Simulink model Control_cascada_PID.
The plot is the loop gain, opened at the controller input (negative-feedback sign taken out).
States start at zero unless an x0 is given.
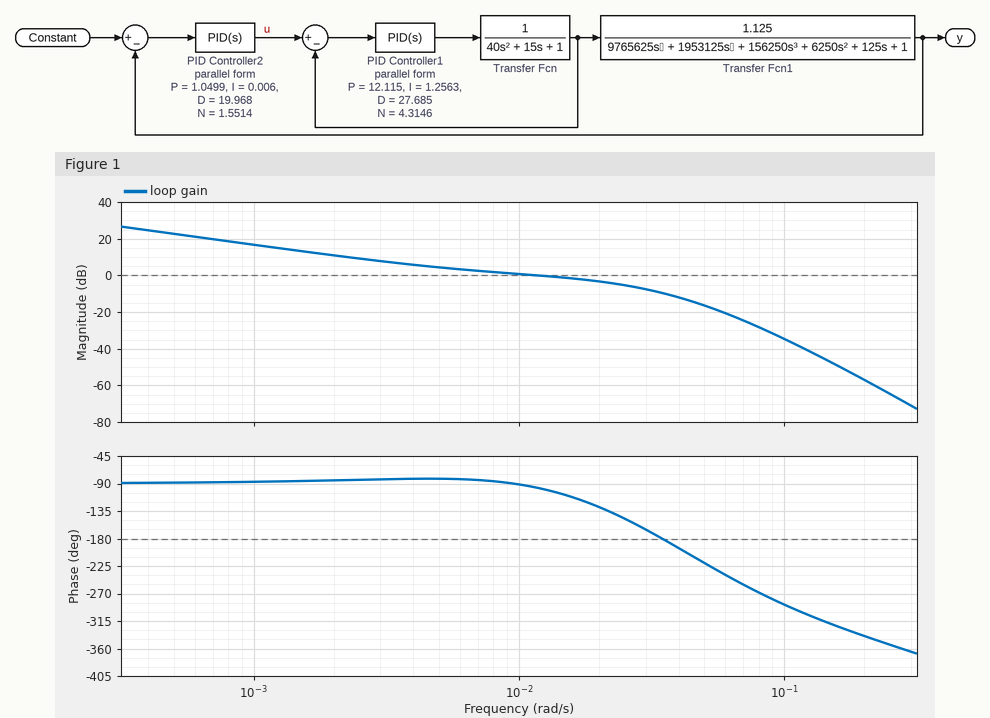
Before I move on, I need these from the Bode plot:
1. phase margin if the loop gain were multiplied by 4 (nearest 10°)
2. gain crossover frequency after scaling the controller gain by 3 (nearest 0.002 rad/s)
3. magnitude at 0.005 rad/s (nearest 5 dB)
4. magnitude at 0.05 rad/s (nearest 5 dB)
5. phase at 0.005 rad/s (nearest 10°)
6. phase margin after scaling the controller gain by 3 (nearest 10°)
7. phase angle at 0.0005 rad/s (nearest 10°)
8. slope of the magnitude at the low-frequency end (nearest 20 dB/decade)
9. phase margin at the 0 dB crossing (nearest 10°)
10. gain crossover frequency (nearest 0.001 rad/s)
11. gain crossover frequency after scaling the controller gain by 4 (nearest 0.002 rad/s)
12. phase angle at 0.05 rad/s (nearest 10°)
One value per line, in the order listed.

-20°
0.034 rad/s
5 dB
-15 dB
-80°
0°
-90°
-20 dB/decade
80°
0.012 rad/s
0.040 rad/s
-220°
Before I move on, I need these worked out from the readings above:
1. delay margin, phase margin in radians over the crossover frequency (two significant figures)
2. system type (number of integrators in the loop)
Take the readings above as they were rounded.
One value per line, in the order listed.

120 s
1
